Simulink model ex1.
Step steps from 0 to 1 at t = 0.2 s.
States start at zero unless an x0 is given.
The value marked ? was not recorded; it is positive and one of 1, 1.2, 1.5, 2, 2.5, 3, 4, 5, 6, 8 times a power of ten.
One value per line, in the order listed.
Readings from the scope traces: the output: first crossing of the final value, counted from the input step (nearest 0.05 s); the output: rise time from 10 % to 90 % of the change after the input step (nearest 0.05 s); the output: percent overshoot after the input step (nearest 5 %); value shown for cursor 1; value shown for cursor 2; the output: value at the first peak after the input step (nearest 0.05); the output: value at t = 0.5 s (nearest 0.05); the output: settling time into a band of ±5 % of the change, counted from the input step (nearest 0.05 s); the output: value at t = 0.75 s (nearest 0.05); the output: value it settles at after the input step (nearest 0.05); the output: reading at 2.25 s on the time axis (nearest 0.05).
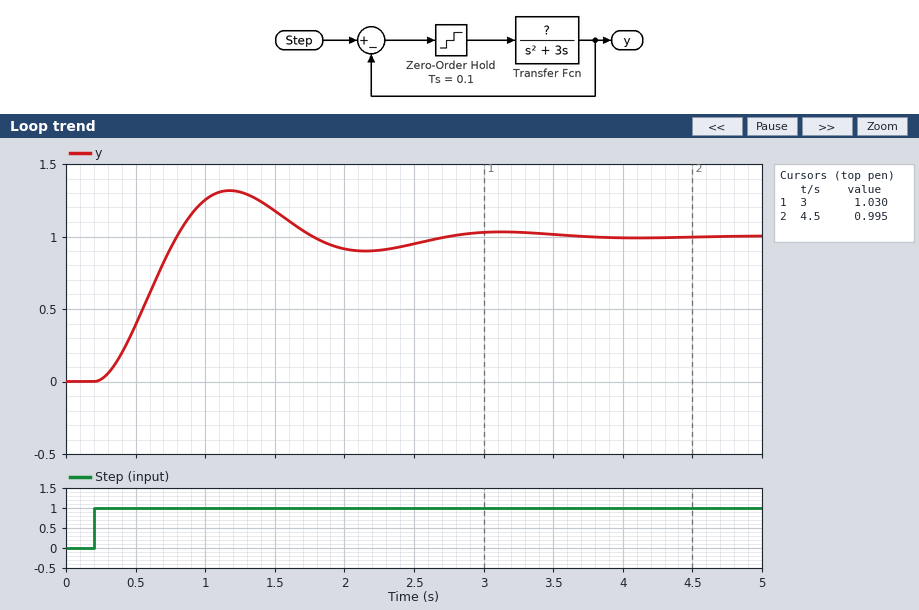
0.60 s
0.40 s
30 %
1.030
0.995
1.30
0.40
2.30 s
0.90
1.00
0.90
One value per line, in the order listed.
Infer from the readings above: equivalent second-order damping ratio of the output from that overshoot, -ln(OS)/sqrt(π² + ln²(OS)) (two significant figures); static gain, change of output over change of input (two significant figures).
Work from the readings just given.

0.36
1.0
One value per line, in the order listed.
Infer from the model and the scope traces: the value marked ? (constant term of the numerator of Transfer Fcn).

12
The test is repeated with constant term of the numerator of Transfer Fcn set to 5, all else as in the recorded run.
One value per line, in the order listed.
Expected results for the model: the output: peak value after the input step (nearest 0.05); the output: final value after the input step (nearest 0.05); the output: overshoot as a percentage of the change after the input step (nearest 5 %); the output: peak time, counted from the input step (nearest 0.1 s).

1.10
1.00
10 %
1.8 s
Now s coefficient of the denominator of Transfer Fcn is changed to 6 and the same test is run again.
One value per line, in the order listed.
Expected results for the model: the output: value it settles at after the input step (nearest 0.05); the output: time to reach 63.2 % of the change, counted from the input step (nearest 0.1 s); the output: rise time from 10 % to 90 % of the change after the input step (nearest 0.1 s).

1.00
0.5 s
0.7 s
